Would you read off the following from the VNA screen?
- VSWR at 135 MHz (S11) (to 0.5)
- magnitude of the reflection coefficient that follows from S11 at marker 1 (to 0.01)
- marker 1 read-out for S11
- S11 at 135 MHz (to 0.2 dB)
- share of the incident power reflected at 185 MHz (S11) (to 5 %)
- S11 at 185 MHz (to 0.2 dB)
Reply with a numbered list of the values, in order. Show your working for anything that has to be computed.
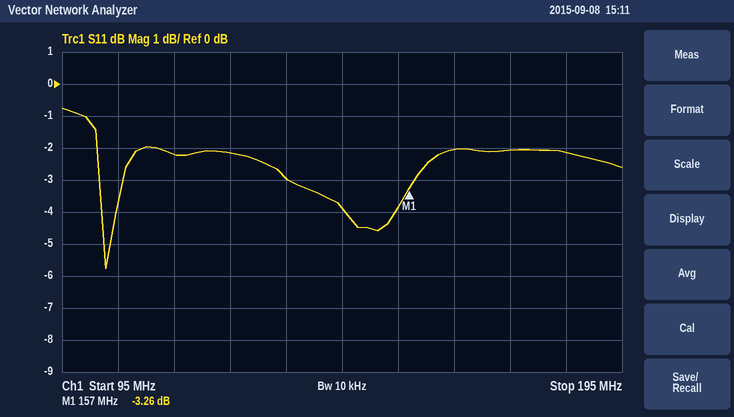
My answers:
1. |Γ| = 10^(-3/20) = 0.7079; VSWR = (1 + 0.7079)/(1 − 0.7079) ≈ 5.85, so 6.0 to the nearest 0.5
2. 10^(-3.26/20) ≈ 0.69
3. -3.26 dB
4. -3.0 dB
5. 10^(-2.2/10) ≈ 60 %
6. -2.2 dB
